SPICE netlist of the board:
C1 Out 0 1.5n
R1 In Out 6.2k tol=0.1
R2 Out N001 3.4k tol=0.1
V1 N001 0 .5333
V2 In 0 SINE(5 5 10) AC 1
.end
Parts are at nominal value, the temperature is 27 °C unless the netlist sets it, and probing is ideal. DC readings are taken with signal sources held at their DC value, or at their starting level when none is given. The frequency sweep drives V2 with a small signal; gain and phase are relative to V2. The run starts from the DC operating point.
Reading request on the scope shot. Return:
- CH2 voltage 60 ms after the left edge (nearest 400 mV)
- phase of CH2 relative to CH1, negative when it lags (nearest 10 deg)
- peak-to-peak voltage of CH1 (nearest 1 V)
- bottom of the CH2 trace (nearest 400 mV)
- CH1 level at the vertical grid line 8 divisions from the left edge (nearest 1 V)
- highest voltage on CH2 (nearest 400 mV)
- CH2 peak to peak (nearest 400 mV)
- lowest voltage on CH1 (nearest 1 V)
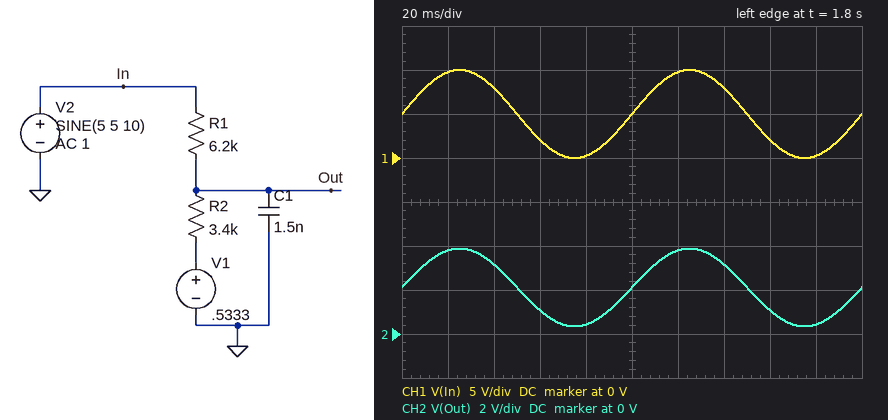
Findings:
1.2 V
0 deg
10 V
400 mV
2 V
4.0 V
3.6 V
0 V
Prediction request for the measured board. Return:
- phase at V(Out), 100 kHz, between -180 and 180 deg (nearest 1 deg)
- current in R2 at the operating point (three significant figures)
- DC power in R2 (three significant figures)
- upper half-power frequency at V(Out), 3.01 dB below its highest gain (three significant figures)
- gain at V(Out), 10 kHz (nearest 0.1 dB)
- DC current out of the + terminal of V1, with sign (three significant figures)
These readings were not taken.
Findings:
-64 deg
465 µA
736 µW
48.3 kHz
-9.2 dB
-465 µA
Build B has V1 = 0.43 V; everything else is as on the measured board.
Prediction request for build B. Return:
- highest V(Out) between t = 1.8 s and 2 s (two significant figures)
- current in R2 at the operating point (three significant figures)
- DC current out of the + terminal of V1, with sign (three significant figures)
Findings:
3.8 V
476 µA
-476 µA
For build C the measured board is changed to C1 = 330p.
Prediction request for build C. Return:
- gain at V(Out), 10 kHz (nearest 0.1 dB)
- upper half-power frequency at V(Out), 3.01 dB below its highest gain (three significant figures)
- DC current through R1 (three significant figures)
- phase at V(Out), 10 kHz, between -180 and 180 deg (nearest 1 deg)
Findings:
-9.0 dB
220 kHz
465 µA
-3 deg
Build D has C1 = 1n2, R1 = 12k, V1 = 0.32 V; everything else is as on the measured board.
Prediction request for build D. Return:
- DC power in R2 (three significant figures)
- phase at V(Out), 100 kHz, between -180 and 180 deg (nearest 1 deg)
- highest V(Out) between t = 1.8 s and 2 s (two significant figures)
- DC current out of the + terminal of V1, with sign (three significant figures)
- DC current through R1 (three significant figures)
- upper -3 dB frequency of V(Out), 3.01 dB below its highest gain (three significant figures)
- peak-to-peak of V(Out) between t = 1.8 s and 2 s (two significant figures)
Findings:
314 µW
-63 deg
2.5 V
-304 µA
304 µA
50.1 kHz
2.2 V
